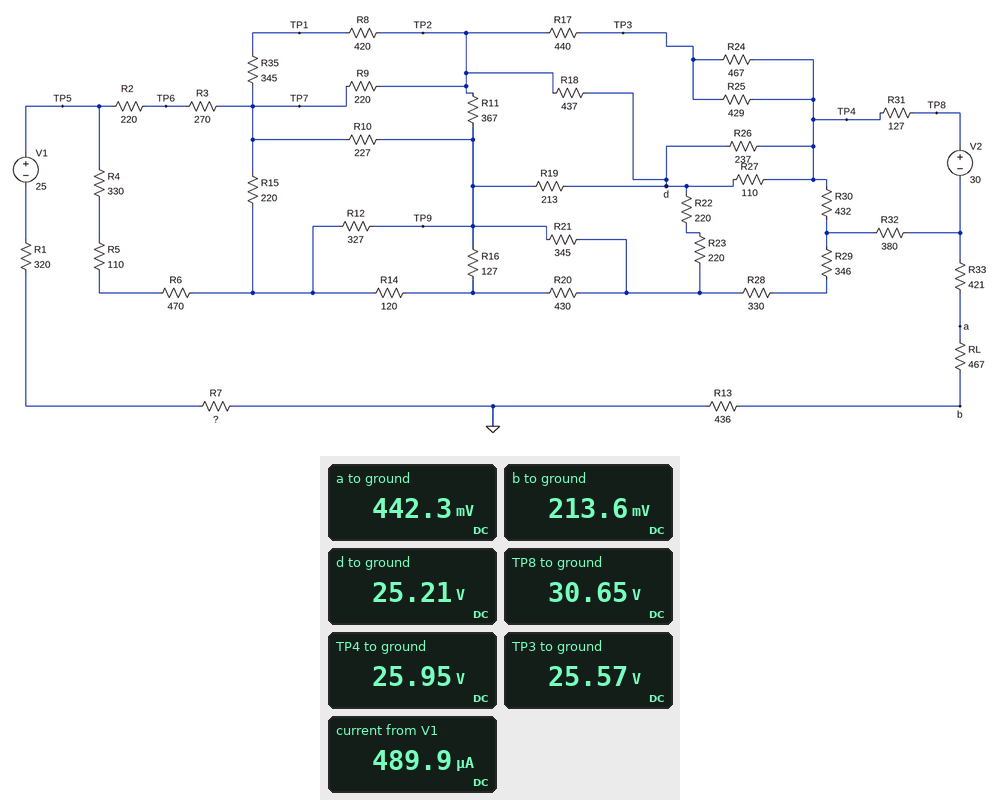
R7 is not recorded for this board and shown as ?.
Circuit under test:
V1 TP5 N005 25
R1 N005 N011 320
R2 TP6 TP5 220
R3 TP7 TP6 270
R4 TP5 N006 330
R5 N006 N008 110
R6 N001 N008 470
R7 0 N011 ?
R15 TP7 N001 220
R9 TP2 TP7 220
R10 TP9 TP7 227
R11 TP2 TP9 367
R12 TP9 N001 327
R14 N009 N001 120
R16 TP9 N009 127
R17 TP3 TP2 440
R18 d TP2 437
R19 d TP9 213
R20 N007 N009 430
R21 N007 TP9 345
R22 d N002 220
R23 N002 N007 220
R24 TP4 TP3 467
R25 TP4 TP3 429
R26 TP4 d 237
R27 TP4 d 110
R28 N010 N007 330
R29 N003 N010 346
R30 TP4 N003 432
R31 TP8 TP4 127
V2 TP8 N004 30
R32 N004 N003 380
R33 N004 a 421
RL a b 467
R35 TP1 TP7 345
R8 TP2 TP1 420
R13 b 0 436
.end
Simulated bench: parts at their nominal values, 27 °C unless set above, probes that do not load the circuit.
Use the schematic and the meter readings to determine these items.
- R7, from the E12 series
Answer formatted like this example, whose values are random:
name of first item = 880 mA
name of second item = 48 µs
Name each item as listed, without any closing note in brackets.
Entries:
R7, from the E12 series = 390 Ω
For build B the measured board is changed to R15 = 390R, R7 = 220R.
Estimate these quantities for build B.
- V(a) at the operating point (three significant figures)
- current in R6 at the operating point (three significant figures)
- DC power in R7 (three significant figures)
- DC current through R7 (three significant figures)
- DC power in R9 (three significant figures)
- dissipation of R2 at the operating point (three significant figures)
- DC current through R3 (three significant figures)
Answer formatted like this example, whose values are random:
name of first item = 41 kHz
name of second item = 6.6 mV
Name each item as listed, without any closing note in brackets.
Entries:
V(a) at the operating point = 471 mV
current in R6 at the operating point = 366 µA
DC power in R7 = 59.9 µW
DC current through R7 = 522 µA
DC power in R9 = 251 µW
dissipation of R2 at the operating point = 5.33 µW
DC current through R3 = 156 µA
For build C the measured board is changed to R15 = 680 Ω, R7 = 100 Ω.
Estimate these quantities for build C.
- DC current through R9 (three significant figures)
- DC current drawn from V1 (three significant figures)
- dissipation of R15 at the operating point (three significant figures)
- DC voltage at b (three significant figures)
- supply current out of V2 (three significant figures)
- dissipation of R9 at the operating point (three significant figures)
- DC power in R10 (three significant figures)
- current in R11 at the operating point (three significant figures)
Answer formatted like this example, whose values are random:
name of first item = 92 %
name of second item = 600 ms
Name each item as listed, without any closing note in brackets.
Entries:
DC current through R9 = 1.01 mA
DC current drawn from V1 = 547 µA
dissipation of R15 at the operating point = 137 µW
DC voltage at b = 238 mV
supply current out of V2 = 37.0 mA
dissipation of R9 at the operating point = 223 µW
DC power in R10 = 221 µW
current in R11 at the operating point = 1.21 mA
